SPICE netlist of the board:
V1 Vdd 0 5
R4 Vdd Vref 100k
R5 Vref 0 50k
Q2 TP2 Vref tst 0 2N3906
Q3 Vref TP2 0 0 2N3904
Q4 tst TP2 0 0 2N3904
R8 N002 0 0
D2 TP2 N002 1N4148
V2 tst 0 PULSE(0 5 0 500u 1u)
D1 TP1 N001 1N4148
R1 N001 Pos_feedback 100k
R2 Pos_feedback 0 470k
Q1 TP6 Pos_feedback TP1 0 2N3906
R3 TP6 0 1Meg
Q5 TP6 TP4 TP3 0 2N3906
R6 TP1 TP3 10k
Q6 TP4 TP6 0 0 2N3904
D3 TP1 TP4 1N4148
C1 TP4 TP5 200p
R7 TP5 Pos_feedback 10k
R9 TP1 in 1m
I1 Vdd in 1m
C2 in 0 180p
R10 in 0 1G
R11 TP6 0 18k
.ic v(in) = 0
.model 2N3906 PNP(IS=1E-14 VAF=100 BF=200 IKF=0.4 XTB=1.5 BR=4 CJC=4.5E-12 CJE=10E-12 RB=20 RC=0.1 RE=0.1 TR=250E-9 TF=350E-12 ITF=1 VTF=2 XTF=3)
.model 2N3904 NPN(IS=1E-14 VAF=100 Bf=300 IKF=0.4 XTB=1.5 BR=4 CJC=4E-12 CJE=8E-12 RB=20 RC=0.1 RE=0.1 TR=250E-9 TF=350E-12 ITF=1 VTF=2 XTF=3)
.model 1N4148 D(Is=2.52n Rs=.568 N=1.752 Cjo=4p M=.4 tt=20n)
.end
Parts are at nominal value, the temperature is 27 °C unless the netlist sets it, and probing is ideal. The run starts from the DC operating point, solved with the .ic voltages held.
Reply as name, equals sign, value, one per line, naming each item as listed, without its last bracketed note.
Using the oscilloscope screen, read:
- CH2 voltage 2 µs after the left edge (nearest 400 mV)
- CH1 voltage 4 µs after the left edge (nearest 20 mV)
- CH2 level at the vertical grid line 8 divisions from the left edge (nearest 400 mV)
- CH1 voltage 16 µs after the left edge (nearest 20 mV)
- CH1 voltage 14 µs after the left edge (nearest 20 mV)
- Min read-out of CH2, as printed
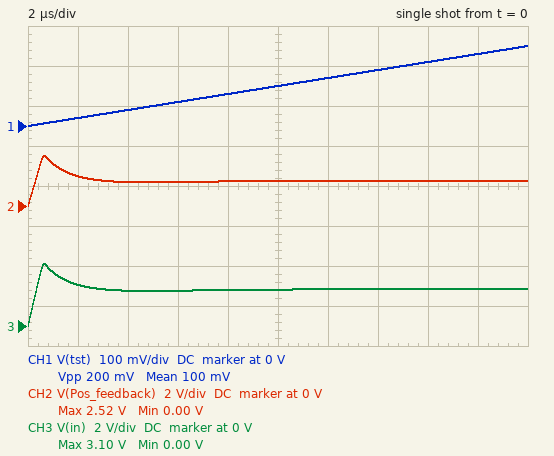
CH2 voltage 2 µs after the left edge = 1.6 V
CH1 voltage 4 µs after the left edge = 40 mV
CH2 level at the vertical grid line 8 divisions from the left edge = 1.2 V
CH1 voltage 16 µs after the left edge = 160 mV
CH1 voltage 14 µs after the left edge = 140 mV
Min read-out of CH2, as printed = 0.00 V
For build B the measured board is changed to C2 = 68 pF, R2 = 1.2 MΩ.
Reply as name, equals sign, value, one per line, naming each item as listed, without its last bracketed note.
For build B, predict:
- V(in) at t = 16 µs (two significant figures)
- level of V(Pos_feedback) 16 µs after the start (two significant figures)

V(in) at t = 16 µs = 3.8 V
level of V(Pos_feedback) 16 µs after the start = 3.2 V
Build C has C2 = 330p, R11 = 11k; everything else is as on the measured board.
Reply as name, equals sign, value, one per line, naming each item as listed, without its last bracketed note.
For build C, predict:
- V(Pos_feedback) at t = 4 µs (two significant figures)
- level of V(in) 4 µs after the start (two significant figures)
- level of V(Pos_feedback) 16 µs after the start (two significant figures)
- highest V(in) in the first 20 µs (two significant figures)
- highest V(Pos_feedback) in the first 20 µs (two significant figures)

V(Pos_feedback) at t = 4 µs = 1.0 V
level of V(in) 4 µs after the start = 1.6 V
level of V(Pos_feedback) 16 µs after the start = 1.4 V
highest V(in) in the first 20 µs = 5.4 V
highest V(Pos_feedback) in the first 20 µs = 4.8 V
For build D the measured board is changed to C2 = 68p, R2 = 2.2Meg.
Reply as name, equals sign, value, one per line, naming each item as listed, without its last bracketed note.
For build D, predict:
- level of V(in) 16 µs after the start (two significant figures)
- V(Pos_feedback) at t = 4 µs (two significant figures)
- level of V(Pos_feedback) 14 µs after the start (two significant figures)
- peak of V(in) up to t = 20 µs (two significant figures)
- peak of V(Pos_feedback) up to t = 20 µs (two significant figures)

level of V(in) 16 µs after the start = 6.2 V
V(Pos_feedback) at t = 4 µs = 3.5 V
level of V(Pos_feedback) 14 µs after the start = 5.5 V
peak of V(in) up to t = 20 µs = 6.4 V
peak of V(Pos_feedback) up to t = 20 µs = 5.8 V
